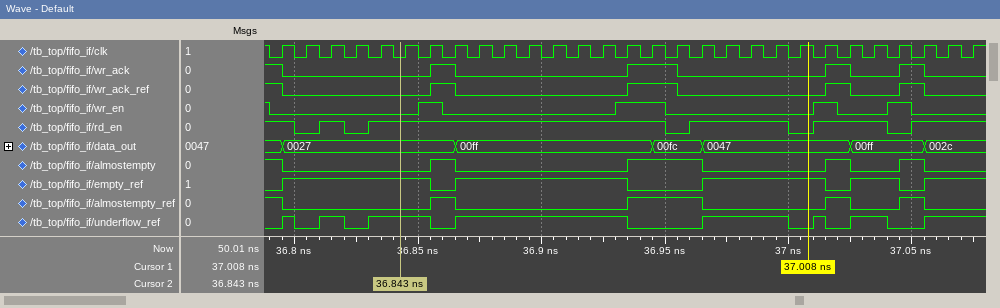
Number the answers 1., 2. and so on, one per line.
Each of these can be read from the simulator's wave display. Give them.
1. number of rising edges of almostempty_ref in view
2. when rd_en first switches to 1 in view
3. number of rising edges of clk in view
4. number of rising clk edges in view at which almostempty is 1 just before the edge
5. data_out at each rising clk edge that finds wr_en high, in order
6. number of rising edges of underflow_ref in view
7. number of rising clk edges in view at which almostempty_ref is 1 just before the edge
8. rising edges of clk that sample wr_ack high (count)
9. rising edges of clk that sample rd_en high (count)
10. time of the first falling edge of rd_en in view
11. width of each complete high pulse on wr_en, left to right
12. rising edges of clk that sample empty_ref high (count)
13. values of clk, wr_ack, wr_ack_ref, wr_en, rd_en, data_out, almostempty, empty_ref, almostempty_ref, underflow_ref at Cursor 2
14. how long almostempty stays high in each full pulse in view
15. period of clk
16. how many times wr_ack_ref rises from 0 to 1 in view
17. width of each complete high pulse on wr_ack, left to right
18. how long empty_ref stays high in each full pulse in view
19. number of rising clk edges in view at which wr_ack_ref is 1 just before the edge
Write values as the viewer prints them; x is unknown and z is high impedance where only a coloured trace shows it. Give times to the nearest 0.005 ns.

1. 4
2. 36.81 ns
3. 29
4. 7
5. 0027, 00ff, 00ff, 0047, 00ff
6. 8
7. 7
8. 6
9. 24
10. 36.8 ns
11. 0.01 ns, 0.02 ns, 0.01 ns, 0.01 ns
12. 22
13. clk=0, wr_ack=0, wr_ack_ref=0, wr_en=0, rd_en=1, data_out=0027, almostempty=0, empty_ref=1, almostempty_ref=0, underflow_ref=1
14. 0.01 ns, 0.03 ns, 0.01 ns, 0.01 ns
15. 0.01 ns
16. 4
17. 0.01 ns, 0.02 ns, 0.01 ns, 0.01 ns
18. 0.06 ns, 0.07 ns, 0.05 ns, 0.02 ns
19. 6
